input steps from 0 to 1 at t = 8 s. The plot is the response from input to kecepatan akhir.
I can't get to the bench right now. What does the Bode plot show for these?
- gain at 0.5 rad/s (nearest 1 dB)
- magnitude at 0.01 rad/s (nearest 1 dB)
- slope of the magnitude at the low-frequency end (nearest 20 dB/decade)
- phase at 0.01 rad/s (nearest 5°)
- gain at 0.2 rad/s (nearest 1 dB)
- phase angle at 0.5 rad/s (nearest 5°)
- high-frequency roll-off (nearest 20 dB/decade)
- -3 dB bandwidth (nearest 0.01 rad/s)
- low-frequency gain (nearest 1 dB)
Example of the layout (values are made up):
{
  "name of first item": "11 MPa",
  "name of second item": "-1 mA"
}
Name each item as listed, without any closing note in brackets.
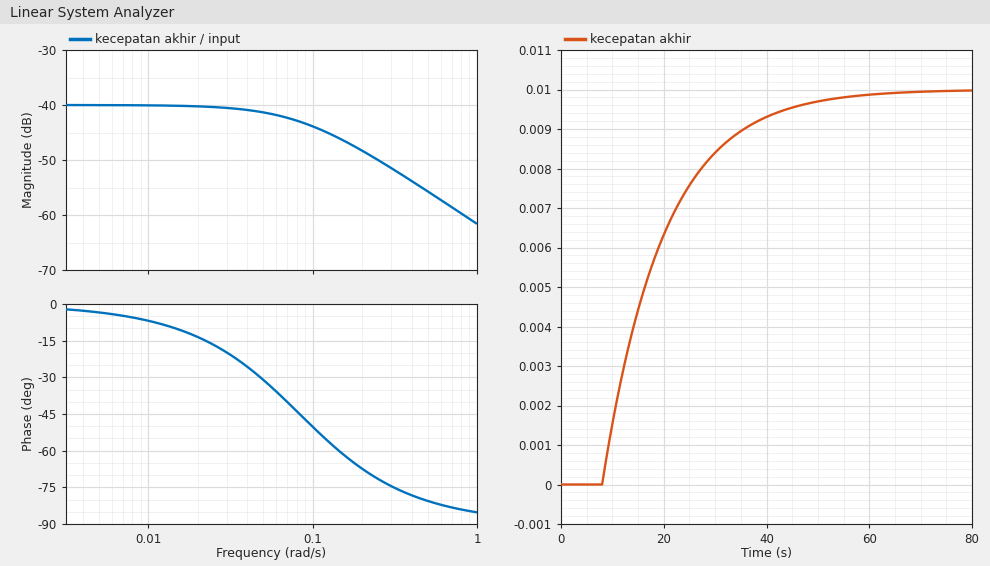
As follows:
{
  "gain at 0.5 rad/s": "-56 dB",
  "magnitude at 0.01 rad/s": "-40 dB",
  "slope of the magnitude at the low-frequency end": "0 dB/decade",
  "phase at 0.01 rad/s": "-5°",
  "gain at 0.2 rad/s": "-48 dB",
  "phase angle at 0.5 rad/s": "-80°",
  "high-frequency roll-off": "-20 dB/decade",
  "-3 dB bandwidth": "0.08 rad/s",
  "low-frequency gain": "-40 dB"
}
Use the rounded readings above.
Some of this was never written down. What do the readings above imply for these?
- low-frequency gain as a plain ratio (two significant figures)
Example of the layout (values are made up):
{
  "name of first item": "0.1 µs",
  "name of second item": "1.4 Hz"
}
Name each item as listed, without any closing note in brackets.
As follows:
{
  "low-frequency gain as a plain ratio": "0.010"
}
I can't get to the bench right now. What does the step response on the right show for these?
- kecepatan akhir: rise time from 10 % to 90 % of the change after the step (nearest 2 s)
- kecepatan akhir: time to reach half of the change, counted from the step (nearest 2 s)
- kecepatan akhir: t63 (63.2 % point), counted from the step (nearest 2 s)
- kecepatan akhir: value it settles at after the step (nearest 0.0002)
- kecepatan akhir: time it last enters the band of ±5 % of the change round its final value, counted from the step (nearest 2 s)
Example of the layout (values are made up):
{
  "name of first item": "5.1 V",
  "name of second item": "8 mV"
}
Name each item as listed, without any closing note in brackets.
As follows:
{
  "kecepatan akhir: rise time from 10 % to 90 % of the change after the step": "26 s",
  "kecepatan akhir: time to reach half of the change, counted from the step": "8 s",
  "kecepatan akhir: t63 (63.2 % point), counted from the step": "12 s",
  "kecepatan akhir: value it settles at after the step": "0.0100",
  "kecepatan akhir: time it last enters the band of ±5 % of the change round its final value, counted from the step": "36 s"
}
